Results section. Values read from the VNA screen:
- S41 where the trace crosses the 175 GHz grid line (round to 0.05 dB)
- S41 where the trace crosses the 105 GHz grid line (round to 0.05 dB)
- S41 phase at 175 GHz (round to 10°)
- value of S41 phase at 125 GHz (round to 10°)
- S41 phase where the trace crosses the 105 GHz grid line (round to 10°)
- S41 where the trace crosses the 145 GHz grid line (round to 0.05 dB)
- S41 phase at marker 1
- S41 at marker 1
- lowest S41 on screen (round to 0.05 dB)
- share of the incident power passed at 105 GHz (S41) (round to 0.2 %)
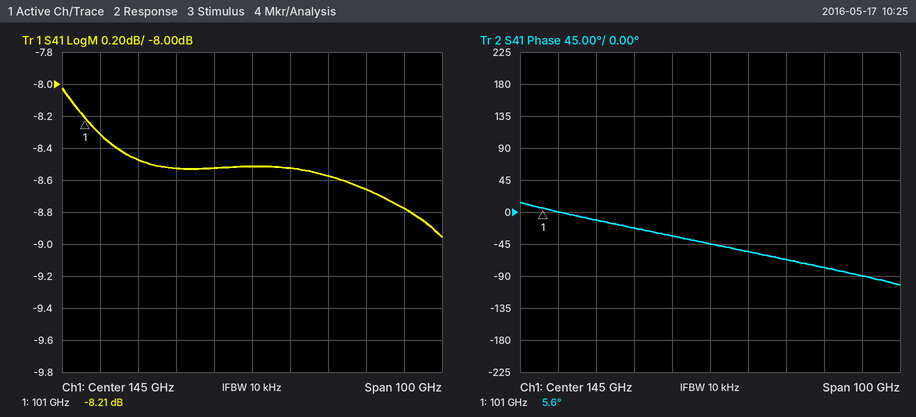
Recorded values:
-8.65 dB
-8.30 dB
-80°
-20°
0°
-8.50 dB
5.6°
-8.21 dB
-8.95 dB
14.8 %
